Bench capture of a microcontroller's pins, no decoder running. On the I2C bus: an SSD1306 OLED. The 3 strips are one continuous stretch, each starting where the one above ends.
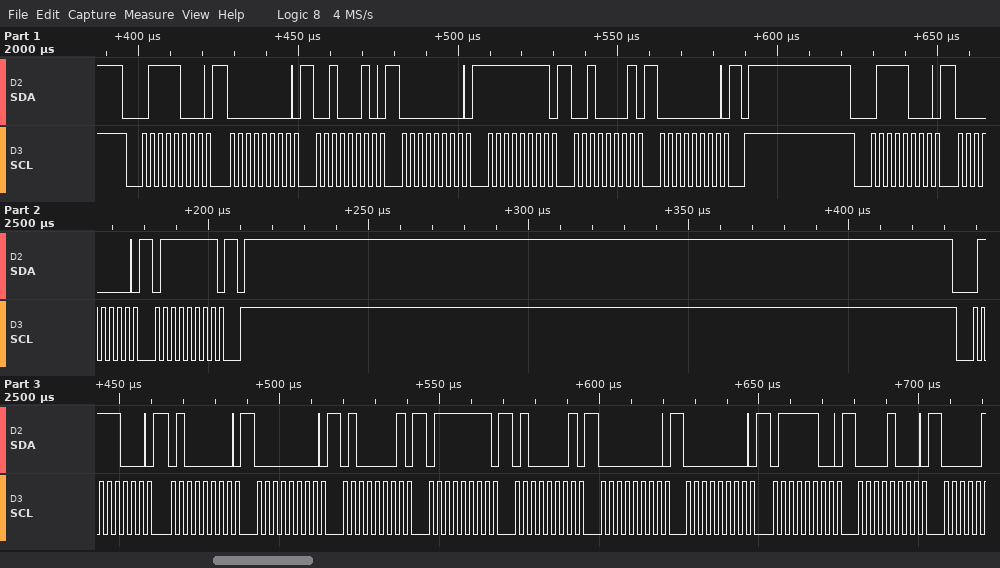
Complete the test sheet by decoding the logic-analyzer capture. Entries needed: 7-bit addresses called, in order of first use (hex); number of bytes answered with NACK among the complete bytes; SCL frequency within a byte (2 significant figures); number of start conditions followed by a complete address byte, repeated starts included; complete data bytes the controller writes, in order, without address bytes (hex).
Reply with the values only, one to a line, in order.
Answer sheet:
0x3C
0
400 kHz
3
00 22 00 FF 21 00 00 7F 40 00 41 7F 41 00 00 7C 08
